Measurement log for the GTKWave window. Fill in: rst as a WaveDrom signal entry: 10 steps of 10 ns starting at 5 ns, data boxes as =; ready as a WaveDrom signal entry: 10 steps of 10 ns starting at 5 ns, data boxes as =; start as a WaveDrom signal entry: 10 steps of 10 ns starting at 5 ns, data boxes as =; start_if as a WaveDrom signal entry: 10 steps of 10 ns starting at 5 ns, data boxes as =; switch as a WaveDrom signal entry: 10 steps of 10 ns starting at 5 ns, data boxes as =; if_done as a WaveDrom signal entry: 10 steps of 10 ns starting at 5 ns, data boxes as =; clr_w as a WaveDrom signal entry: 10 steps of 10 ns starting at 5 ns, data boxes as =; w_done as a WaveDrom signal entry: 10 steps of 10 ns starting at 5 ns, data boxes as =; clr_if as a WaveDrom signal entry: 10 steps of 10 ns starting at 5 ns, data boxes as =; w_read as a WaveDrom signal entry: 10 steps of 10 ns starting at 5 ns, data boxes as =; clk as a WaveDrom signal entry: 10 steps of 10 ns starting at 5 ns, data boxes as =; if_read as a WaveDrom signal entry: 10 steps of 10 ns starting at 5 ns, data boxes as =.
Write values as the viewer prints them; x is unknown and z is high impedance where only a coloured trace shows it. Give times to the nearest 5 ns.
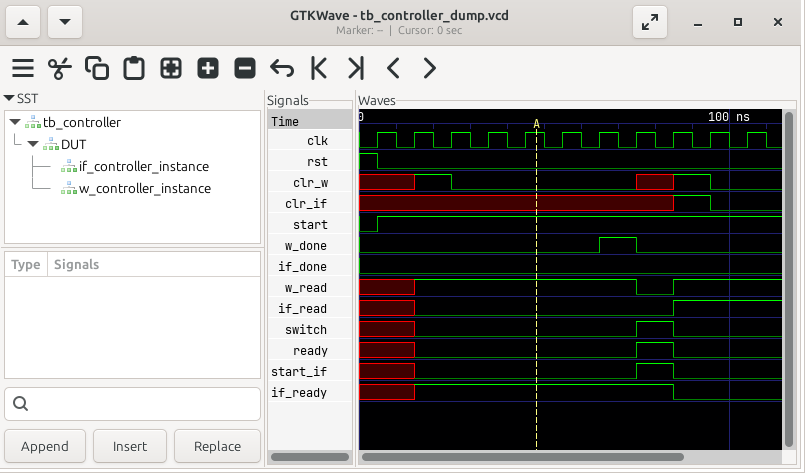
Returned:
{name: 'rst', wave: '0.........'}
{name: 'ready', wave: 'x0.....10.'}
{name: 'start', wave: '1.........'}
{name: 'start_if', wave: 'x0.....10.'}
{name: 'switch', wave: 'x0.....10.'}
{name: 'if_done', wave: '0.........'}
{name: 'clr_w', wave: 'x10....x10'}
{name: 'w_done', wave: '0.....10..'}
{name: 'clr_if', wave: 'x.......10'}
{name: 'w_read', wave: 'x1.....01.'}
{name: 'clk', wave: 'p.........'}
{name: 'if_read', wave: 'x0......1.'}
